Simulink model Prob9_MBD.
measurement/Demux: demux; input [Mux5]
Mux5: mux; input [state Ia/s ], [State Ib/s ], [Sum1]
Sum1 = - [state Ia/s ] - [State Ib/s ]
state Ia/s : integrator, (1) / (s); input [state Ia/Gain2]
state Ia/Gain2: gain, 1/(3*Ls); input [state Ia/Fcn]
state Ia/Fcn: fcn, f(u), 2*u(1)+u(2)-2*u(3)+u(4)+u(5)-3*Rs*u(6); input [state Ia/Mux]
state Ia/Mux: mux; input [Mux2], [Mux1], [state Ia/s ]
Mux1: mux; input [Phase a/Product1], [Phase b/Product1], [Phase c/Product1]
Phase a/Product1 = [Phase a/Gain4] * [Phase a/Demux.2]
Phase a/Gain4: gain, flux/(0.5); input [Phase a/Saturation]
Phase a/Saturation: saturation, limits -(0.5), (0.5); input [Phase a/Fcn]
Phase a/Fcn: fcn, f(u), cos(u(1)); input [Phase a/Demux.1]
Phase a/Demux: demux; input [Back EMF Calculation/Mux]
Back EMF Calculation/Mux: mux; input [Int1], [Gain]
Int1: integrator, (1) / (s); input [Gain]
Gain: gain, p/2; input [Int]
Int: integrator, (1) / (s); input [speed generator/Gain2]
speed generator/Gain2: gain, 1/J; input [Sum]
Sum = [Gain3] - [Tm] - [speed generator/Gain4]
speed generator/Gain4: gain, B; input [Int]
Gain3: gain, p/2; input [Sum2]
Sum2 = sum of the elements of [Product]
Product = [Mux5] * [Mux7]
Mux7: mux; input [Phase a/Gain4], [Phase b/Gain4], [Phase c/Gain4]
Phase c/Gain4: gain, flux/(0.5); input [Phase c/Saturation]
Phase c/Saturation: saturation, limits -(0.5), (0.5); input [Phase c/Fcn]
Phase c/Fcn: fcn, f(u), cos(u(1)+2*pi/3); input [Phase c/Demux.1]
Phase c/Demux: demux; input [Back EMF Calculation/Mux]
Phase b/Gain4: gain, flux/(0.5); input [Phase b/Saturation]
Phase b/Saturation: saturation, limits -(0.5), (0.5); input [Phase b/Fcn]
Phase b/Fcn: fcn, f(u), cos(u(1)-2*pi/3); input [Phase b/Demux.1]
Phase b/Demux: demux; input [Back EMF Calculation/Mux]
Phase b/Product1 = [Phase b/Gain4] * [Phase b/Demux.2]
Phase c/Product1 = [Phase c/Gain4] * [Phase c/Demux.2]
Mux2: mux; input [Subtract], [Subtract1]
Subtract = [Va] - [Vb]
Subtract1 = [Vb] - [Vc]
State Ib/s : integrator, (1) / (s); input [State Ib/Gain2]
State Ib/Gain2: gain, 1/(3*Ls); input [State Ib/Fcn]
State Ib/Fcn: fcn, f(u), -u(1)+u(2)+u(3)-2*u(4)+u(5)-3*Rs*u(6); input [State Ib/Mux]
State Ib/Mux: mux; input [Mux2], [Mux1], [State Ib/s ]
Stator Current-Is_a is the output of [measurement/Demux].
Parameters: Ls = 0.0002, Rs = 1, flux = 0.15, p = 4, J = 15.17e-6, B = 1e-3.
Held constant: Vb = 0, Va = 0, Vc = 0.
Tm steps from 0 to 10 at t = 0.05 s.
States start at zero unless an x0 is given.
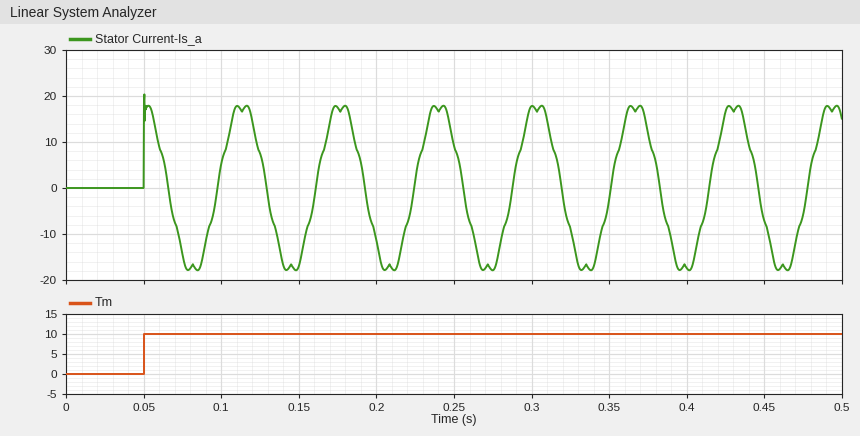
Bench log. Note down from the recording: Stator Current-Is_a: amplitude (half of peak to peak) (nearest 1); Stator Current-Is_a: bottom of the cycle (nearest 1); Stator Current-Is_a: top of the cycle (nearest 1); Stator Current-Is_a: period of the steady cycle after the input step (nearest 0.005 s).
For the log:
18
-18
18
0.065 s
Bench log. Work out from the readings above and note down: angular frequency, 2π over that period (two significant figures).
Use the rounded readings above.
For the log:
97 rad/s
